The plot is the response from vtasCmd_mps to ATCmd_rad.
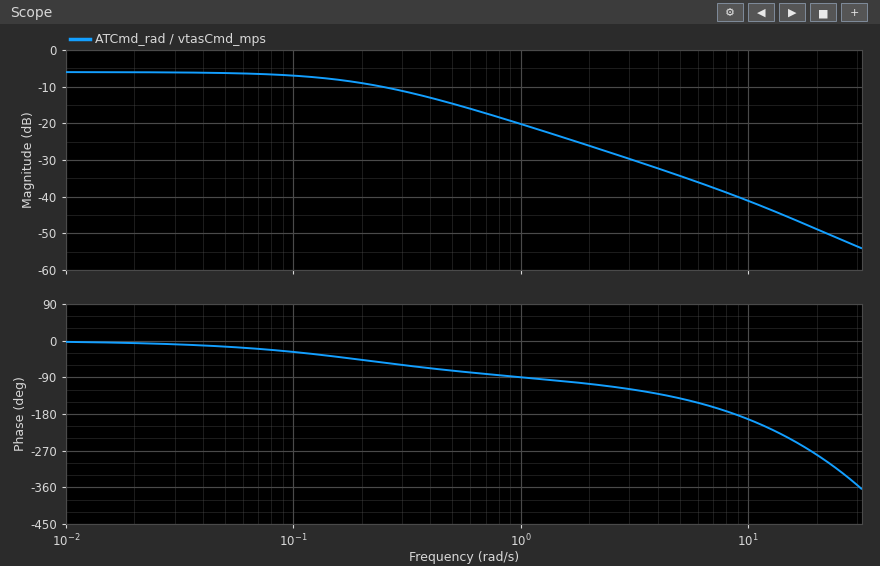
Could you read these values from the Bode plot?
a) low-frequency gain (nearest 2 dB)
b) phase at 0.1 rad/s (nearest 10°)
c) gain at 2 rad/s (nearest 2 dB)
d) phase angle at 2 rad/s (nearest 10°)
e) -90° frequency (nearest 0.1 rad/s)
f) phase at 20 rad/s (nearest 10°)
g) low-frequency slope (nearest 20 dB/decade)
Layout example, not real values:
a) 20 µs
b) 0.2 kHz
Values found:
a) -6 dB
b) -30°
c) -26 dB
d) -110°
e) 1.0 rad/s
f) -280°
g) 0 dB/decade
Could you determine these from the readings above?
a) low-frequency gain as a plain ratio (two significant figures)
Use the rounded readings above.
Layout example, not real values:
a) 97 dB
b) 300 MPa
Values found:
a) 0.50
